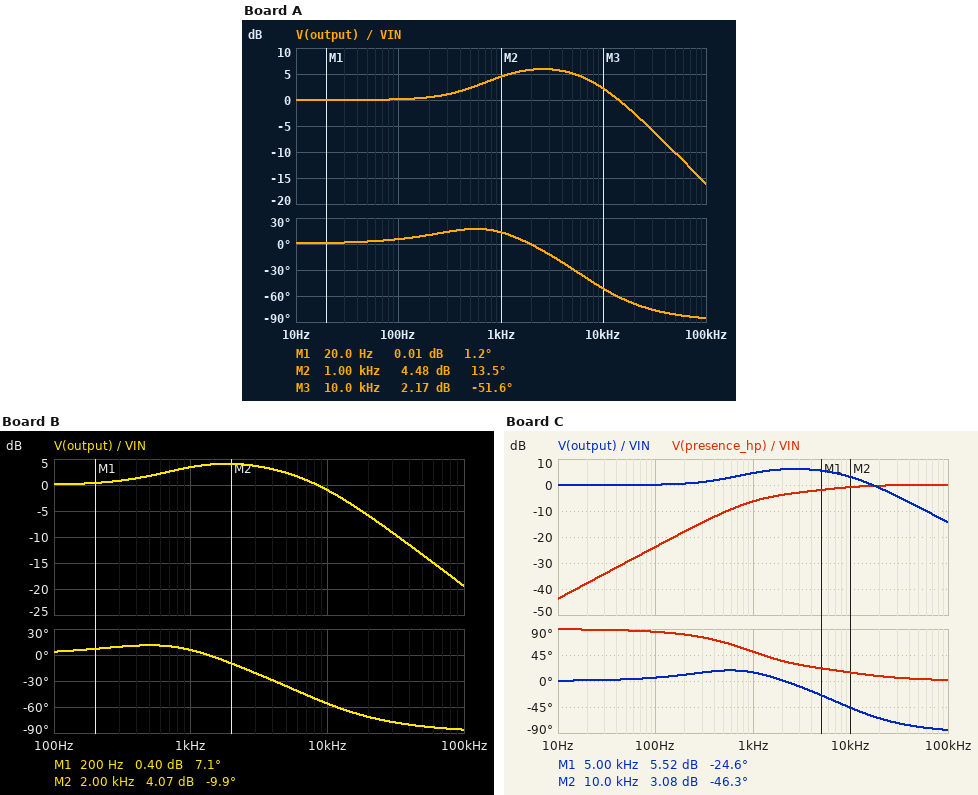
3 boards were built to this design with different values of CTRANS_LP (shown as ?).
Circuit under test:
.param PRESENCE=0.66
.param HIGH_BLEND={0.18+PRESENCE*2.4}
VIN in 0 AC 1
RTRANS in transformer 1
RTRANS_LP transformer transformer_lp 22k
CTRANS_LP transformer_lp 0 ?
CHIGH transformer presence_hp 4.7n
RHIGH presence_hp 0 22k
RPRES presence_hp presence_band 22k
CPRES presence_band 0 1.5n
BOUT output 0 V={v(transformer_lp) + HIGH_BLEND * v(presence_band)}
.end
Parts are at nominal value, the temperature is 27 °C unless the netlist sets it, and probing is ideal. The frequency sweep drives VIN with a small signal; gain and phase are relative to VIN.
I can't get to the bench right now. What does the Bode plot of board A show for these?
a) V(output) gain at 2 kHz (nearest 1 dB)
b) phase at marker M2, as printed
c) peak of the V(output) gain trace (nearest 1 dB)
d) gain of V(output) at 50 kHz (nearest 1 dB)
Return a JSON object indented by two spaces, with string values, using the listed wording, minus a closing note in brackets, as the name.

{
  "V(output) gain at 2 kHz": "6 dB",
  "phase at marker M2, as printed": "13.5 deg",
  "peak of the V(output) gain trace": "6 dB",
  "gain of V(output) at 50 kHz": "-10 dB"
}
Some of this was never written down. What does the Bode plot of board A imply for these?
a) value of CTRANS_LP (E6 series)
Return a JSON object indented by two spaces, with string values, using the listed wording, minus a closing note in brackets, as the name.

{
  "value of CTRANS_LP": "1 nF"
}
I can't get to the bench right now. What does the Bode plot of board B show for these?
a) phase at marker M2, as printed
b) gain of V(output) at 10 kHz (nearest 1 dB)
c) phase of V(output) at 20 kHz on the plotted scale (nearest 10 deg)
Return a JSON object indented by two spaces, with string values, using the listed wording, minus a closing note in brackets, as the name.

{
  "phase at marker M2, as printed": "-9.9 deg",
  "gain of V(output) at 10 kHz": "-1 dB",
  "phase of V(output) at 20 kHz on the plotted scale": "-70 deg"
}
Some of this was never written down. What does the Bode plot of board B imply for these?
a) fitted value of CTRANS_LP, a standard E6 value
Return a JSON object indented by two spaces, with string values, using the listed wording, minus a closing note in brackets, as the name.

{
  "fitted value of CTRANS_LP, a standard E6 value": "3.3 nF"
}
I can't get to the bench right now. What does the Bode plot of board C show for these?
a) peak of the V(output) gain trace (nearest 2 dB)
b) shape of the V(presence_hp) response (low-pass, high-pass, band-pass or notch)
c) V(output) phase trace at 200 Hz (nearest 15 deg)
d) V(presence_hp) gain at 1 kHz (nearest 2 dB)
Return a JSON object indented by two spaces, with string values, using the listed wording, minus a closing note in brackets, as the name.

{
  "peak of the V(output) gain trace": "6 dB",
  "shape of the V(presence_hp) response": "high-pass",
  "V(output) phase trace at 200 Hz": "15 deg",
  "V(presence_hp) gain at 1 kHz": "-6 dB"
}
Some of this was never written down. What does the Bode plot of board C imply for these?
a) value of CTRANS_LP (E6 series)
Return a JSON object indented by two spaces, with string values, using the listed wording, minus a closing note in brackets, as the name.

{
  "value of CTRANS_LP": "680 pF"
}
